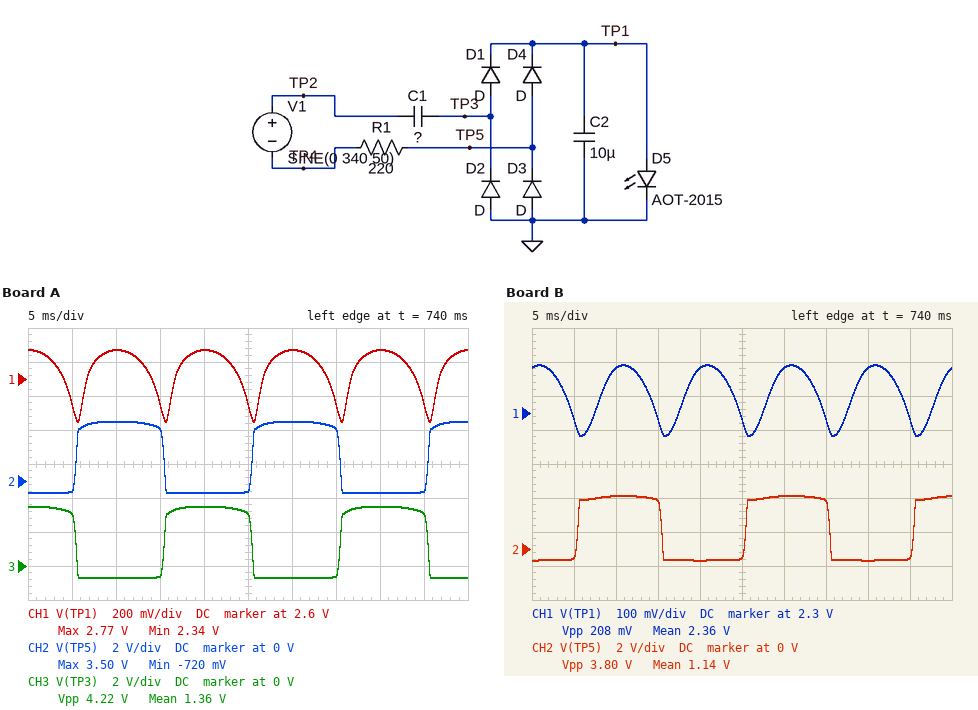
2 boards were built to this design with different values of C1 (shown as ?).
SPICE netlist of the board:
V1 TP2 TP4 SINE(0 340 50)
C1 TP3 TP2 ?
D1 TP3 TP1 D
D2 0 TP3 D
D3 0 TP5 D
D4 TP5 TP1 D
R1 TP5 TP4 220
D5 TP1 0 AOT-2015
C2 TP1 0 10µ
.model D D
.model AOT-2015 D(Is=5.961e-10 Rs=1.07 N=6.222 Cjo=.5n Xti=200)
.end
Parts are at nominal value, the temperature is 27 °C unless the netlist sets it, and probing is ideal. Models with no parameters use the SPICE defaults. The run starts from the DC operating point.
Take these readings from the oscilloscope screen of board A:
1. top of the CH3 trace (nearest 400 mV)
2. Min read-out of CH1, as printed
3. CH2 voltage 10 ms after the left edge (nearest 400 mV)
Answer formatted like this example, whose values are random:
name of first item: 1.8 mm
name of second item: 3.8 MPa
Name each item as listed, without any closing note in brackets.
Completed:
top of the CH3 trace: 3.6 V
Min read-out of CH1, as printed: 2.34 V
CH2 voltage 10 ms after the left edge: 3.6 V
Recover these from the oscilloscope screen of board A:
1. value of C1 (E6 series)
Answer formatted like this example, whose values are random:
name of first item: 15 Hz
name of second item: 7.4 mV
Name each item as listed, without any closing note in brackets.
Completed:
value of C1: 150 nF
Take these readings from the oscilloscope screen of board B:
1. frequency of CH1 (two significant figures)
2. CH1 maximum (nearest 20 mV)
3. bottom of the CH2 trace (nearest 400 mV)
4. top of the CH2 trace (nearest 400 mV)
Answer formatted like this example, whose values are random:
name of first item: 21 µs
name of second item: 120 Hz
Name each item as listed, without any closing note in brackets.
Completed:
frequency of CH1: 100 Hz
CH1 maximum: 2.44 V
bottom of the CH2 trace: -800 mV
top of the CH2 trace: 3.2 V
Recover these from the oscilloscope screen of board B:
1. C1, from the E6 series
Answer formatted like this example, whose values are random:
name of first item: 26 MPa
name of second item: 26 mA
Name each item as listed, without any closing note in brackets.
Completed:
C1, from the E6 series: 22 nF
